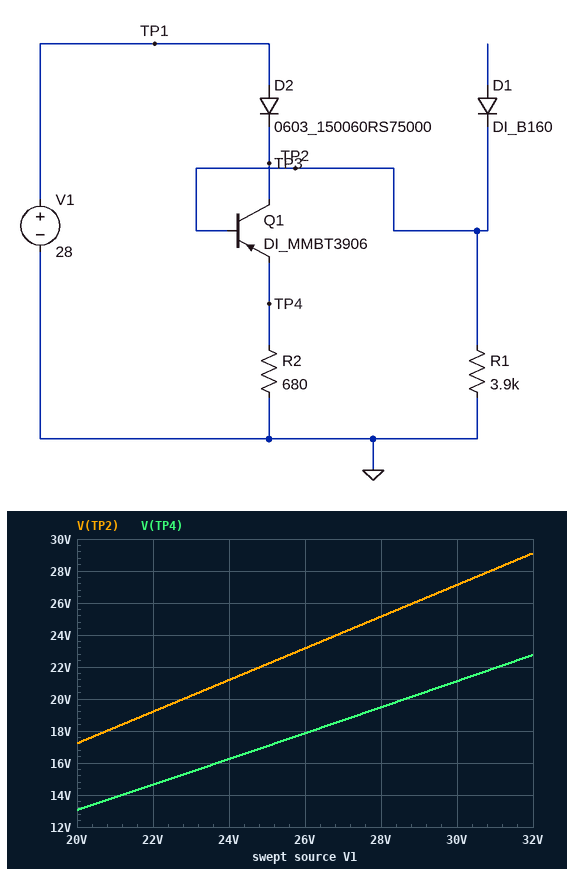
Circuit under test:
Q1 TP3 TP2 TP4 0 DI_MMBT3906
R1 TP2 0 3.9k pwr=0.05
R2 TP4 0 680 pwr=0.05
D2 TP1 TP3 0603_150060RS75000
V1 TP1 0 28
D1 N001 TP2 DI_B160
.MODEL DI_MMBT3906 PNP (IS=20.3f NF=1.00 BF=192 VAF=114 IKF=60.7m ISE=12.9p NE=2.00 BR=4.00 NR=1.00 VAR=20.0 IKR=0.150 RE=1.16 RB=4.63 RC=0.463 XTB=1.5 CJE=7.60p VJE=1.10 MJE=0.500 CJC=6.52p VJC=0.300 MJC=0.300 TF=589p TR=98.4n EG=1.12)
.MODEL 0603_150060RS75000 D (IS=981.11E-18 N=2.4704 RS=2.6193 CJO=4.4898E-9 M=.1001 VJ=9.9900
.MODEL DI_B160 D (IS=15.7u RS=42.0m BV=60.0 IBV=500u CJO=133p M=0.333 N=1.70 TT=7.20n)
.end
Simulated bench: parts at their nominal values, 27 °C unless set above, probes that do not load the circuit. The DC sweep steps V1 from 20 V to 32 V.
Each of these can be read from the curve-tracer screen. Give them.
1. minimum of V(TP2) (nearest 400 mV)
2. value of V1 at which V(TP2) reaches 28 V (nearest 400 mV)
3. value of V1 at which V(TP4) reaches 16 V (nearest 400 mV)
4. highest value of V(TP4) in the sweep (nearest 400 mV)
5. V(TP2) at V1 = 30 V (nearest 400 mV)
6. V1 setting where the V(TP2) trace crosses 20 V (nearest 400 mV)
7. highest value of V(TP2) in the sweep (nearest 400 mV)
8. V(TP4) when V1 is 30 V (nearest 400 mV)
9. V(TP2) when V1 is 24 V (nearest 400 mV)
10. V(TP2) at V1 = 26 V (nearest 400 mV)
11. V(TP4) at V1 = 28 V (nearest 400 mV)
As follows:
17.2 V
30.8 V
23.6 V
22.8 V
27.2 V
22.8 V
29.2 V
21.2 V
21.2 V
23.2 V
19.6 V
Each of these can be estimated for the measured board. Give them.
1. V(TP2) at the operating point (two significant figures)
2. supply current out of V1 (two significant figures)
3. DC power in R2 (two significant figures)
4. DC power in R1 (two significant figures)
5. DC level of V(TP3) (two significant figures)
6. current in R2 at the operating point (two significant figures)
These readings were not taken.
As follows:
25 V
35 mA
560 mW
160 mW
26 V
29 mA
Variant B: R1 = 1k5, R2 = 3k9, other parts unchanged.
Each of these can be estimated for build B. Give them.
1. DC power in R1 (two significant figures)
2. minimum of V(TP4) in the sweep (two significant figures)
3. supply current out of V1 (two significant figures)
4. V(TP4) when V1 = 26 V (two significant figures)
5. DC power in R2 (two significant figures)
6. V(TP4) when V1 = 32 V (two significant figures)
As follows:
420 mW
18 V
23 mA
24 V
170 mW
30 V
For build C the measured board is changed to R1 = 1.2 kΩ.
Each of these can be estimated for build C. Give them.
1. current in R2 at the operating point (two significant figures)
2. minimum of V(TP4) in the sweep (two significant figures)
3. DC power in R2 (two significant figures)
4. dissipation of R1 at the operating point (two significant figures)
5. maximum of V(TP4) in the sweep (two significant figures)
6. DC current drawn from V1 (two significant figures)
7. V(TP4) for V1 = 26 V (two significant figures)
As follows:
38 mA
18 V
970 mW
520 mW
30 V
59 mA
24 V
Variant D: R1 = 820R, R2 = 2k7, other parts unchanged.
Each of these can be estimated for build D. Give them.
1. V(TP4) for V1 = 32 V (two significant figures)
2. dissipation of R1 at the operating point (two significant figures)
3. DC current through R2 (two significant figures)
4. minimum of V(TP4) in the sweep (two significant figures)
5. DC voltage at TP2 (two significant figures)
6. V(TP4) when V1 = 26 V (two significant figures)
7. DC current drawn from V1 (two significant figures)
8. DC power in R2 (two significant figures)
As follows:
30 V
760 mW
9.6 mA
18 V
25 V
24 V
40 mA
250 mW
